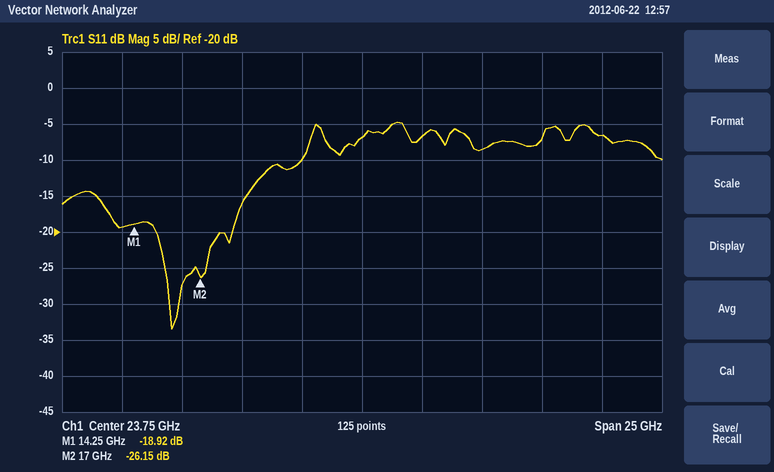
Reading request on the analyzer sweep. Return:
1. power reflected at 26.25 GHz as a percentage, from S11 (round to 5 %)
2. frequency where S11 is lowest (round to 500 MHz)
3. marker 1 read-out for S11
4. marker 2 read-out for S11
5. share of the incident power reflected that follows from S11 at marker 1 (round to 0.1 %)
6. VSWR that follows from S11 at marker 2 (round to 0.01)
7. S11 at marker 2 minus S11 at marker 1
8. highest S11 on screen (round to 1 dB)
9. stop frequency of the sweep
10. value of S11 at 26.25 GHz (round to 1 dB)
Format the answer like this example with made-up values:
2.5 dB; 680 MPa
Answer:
20 %; 16.0 GHz; -18.92 dB; -26.15 dB; 1.3 %; 1.10; -7.23 dB; -5 dB; 36.25 GHz; -7 dB
